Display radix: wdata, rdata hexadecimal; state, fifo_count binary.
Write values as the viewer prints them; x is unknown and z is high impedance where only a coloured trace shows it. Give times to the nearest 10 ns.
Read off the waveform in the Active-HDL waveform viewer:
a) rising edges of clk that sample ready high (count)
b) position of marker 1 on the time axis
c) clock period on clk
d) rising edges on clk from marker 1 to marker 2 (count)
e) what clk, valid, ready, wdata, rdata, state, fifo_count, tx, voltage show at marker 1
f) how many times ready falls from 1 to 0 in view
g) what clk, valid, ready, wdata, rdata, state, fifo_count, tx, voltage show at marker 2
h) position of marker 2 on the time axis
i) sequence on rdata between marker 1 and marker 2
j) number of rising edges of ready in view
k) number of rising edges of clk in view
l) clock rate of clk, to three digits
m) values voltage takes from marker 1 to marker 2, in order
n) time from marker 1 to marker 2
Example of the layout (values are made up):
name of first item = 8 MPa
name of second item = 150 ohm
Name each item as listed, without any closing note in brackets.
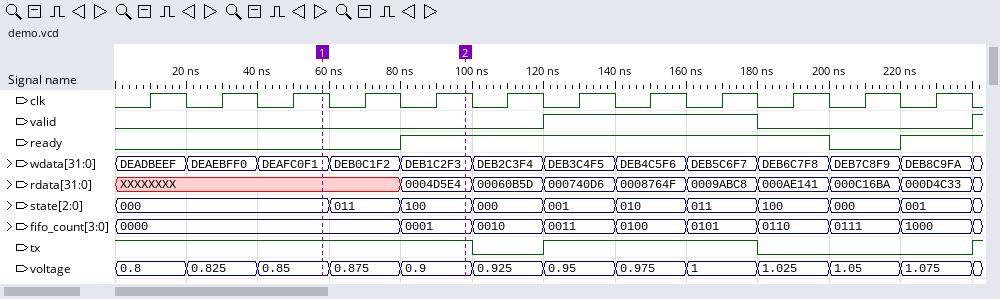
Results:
rising edges of clk that sample ready high = 7
position of marker 1 on the time axis = 60 ns
clock period on clk = 20 ns
rising edges on clk from marker 1 to marker 2 = 2
what clk, valid, ready, wdata, rdata, state, fifo_count, tx, voltage show at marker 1 = clk=1, valid=0, ready=0, wdata=DEAFC0F1, rdata=XXXXXXXX, state=000, fifo_count=0000, tx=1, voltage=0.85
how many times ready falls from 1 to 0 in view = 1
what clk, valid, ready, wdata, rdata, state, fifo_count, tx, voltage show at marker 2 = clk=1, valid=0, ready=1, wdata=DEB1C2F3, rdata=0004D5E4, state=100, fifo_count=0001, tx=1, voltage=0.9
position of marker 2 on the time axis = 100 ns
sequence on rdata between marker 1 and marker 2 = XXXXXXXX, 0004D5E4
number of rising edges of ready in view = 2
number of rising edges of clk in view = 12
clock rate of clk, to three digits = 50.0 MHz
values voltage takes from marker 1 to marker 2, in order = 0.85, 0.875, 0.9
time from marker 1 to marker 2 = 40 ns
